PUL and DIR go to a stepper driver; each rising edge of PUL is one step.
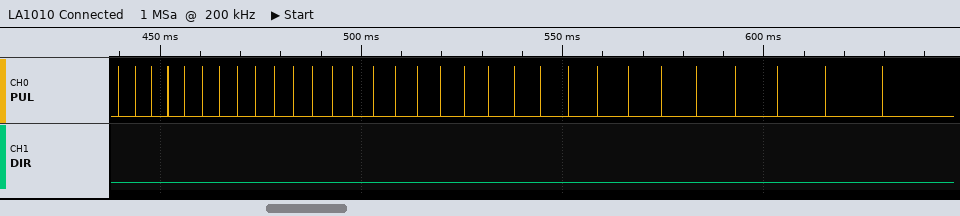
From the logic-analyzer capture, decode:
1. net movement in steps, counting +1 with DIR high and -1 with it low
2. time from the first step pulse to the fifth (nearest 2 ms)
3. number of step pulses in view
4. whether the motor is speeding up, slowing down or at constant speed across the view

-31
16 ms
31
slowing down
